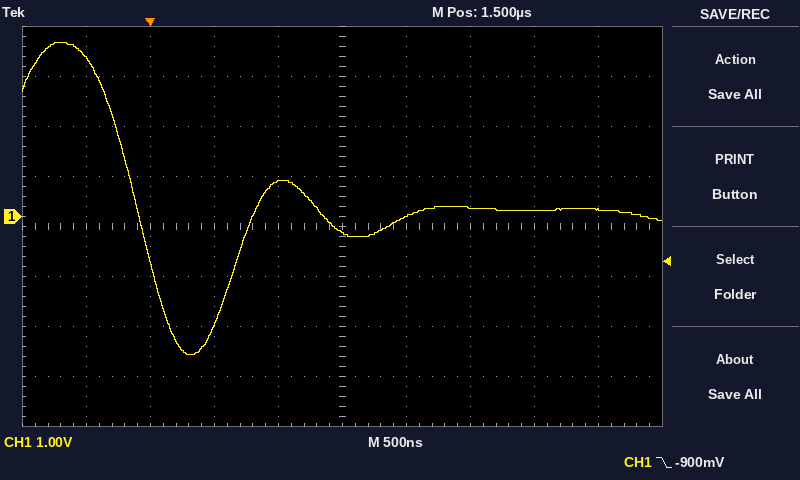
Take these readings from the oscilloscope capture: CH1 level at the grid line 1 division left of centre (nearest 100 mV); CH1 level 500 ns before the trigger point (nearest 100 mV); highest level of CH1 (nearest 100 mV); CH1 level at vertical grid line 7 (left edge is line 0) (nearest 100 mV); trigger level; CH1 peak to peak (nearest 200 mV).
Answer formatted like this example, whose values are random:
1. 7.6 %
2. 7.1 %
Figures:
1. 700 mV
2. 3.2 V
3. 3.5 V
4. 200 mV
5. -900 mV
6. 6.2 V
